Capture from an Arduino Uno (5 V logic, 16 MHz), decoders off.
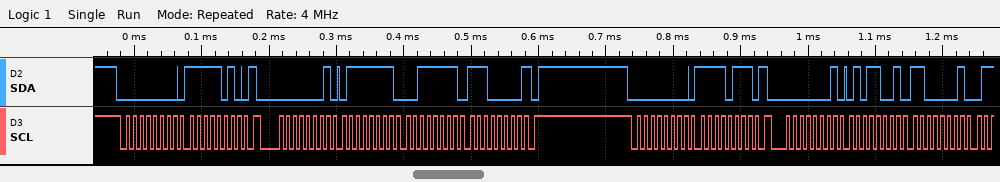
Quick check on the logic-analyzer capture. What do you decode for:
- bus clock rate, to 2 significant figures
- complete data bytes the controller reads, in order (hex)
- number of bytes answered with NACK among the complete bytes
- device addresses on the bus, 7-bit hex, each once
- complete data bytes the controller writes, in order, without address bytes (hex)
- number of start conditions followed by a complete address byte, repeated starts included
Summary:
100 kHz
7F 3F E0 59 C1
1
0x00
FA F7
4
